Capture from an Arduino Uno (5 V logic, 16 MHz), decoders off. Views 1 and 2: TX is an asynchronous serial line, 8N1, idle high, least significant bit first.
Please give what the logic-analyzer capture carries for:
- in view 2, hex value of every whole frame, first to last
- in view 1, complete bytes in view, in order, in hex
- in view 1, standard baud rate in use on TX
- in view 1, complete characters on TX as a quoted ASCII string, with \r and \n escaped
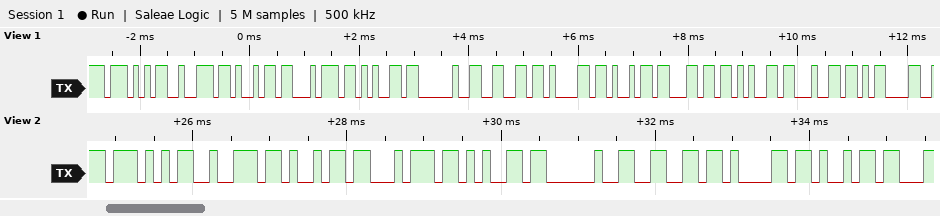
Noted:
57 72 69 74 65 20 66 61 69
57 72 69 74 65 20 66 61 69 6C 65 64 0D
9600 baud
"Write failed\r"
